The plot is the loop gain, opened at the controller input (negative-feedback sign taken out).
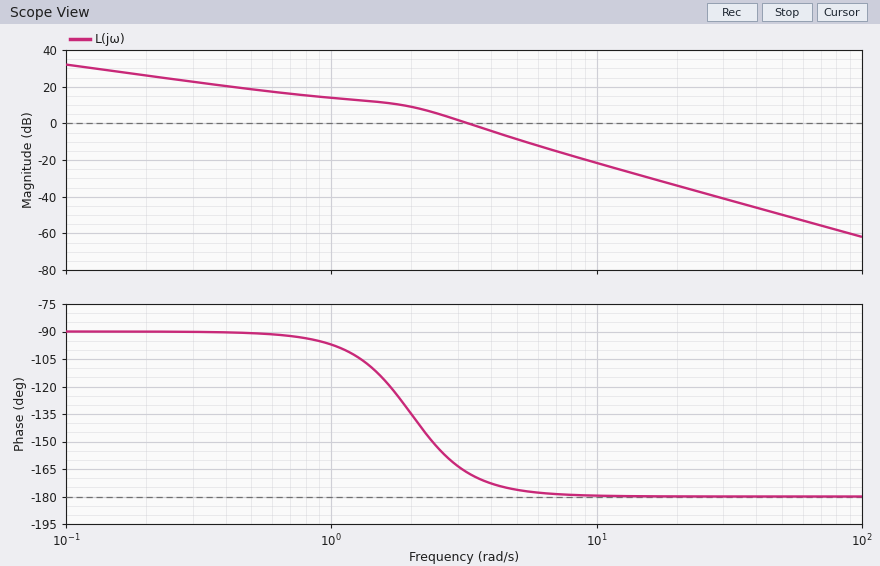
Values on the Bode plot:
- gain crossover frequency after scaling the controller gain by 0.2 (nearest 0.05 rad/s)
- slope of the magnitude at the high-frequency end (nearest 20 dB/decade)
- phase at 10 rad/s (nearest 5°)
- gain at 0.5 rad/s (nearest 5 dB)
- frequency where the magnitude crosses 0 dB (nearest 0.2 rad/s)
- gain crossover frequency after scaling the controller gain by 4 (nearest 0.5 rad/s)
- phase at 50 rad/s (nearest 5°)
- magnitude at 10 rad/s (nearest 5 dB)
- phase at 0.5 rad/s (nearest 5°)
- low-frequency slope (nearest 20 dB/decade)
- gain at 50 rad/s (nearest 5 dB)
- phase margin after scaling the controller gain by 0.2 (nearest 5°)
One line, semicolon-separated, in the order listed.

1.00 rad/s; -40 dB/decade; -180°; 20 dB; 3.2 rad/s; 6.0 rad/s; -180°; -20 dB; -90°; -20 dB/decade; -50 dB; 85°
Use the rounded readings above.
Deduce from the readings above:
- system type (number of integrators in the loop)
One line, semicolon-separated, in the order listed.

1
